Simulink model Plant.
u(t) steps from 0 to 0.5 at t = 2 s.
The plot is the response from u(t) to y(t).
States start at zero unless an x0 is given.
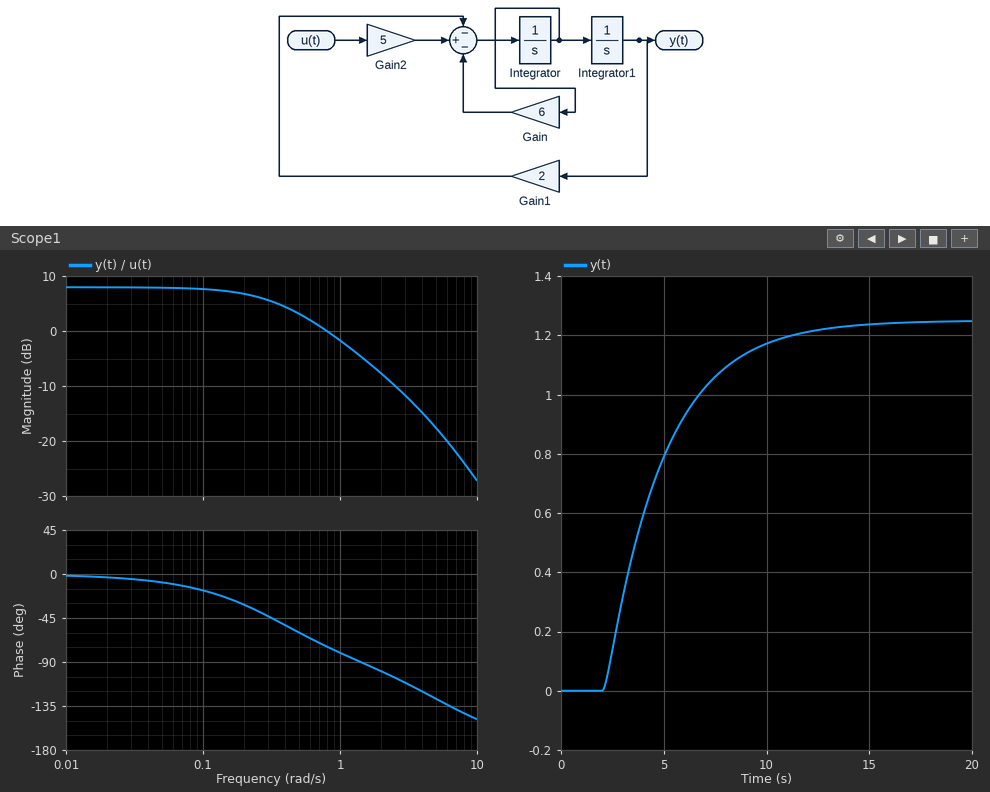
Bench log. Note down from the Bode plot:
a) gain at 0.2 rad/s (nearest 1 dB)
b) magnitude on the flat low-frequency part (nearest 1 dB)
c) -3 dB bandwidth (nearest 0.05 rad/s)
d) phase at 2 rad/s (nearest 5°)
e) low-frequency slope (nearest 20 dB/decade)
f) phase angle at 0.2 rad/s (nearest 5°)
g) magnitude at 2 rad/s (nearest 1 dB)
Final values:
7 dB
8 dB
0.35 rad/s
-100°
0 dB/decade
-30°
-8 dB
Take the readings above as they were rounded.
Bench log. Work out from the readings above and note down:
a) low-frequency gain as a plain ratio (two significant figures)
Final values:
2.5
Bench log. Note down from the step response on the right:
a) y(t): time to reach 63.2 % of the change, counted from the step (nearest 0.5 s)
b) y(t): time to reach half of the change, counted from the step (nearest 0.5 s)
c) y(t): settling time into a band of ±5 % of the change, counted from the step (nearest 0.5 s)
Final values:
3.0 s
2.0 s
8.5 s
